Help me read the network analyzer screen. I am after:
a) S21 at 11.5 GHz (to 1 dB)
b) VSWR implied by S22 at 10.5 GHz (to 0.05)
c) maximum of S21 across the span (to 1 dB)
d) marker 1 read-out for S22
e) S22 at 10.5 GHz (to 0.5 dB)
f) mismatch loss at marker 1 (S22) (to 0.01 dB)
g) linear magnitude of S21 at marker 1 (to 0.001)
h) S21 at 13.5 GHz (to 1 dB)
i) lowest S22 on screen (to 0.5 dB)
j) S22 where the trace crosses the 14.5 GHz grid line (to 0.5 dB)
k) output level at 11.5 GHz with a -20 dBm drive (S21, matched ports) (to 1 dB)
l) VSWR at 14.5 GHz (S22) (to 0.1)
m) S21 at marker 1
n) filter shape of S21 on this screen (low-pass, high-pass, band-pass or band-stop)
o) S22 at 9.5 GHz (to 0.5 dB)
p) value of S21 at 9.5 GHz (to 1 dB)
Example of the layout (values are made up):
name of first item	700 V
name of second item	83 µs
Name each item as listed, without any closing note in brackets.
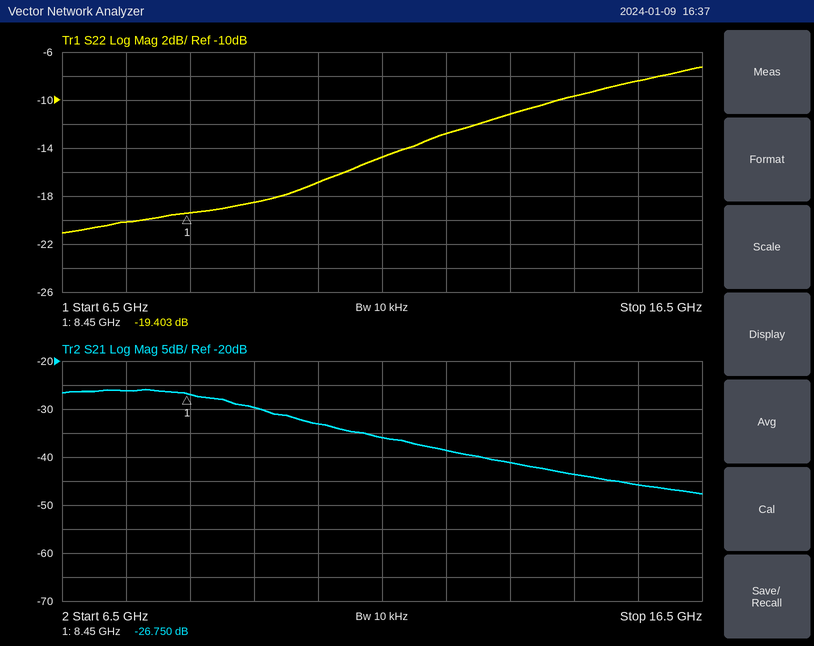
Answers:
S21 at 11.5 GHz	-36 dB
VSWR implied by S22 at 10.5 GHz	1.35
maximum of S21 across the span	-26 dB
marker 1 read-out for S22	-19.403 dB
S22 at 10.5 GHz	-17.0 dB
mismatch loss at marker 1 (S22)	0.05 dB
linear magnitude of S21 at marker 1	0.046
S21 at 13.5 GHz	-41 dB
lowest S22 on screen	-21.0 dB
S22 where the trace crosses the 14.5 GHz grid line	-9.5 dB
output level at 11.5 GHz with a -20 dBm drive (S21, matched ports)	-56 dBm
VSWR at 14.5 GHz (S22)	2.0
S21 at marker 1	-26.750 dB
filter shape of S21 on this screen	low-pass
S22 at 9.5 GHz	-18.5 dB
value of S21 at 9.5 GHz	-30 dB
